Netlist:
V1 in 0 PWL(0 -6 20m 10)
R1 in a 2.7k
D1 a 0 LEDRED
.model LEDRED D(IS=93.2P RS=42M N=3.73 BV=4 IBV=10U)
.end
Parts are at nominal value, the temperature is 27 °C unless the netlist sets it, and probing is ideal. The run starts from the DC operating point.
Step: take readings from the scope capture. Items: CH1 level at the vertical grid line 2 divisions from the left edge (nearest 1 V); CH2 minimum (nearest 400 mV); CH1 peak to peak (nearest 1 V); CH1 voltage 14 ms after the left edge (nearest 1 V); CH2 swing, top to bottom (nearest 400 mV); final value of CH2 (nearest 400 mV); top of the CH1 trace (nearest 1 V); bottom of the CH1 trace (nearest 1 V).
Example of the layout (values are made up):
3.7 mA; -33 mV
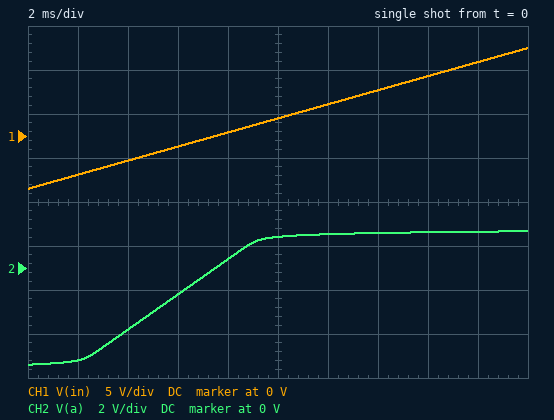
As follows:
-3 V; -4.4 V; 16 V; 5 V; 6.0 V; 1.6 V; 10 V; -6 V
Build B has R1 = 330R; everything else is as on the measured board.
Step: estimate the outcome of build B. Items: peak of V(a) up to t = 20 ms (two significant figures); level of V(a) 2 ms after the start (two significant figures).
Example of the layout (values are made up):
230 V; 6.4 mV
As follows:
1.9 V; -4.3 V
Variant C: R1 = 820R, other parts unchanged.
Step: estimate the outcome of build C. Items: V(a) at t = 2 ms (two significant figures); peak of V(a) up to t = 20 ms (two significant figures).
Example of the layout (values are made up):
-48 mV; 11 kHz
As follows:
-4.3 V; 1.8 V
